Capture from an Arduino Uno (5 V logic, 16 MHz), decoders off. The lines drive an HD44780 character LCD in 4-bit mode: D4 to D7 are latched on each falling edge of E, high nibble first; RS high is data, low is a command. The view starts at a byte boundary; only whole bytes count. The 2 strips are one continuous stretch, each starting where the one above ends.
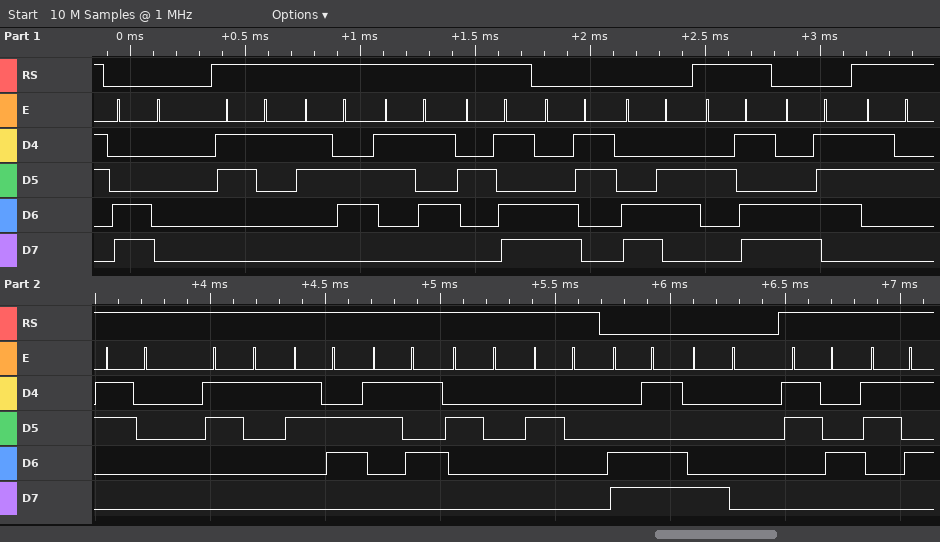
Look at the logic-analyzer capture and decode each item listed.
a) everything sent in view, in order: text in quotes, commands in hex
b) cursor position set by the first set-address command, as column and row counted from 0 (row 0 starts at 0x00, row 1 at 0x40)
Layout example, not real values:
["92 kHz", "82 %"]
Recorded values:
["0xC0 \"165-\" 0xC3 0xC6 \"-\" 0xC7 \"20165  \" 0xCD 0x80 \"45\"", "column 0, row 1"]
